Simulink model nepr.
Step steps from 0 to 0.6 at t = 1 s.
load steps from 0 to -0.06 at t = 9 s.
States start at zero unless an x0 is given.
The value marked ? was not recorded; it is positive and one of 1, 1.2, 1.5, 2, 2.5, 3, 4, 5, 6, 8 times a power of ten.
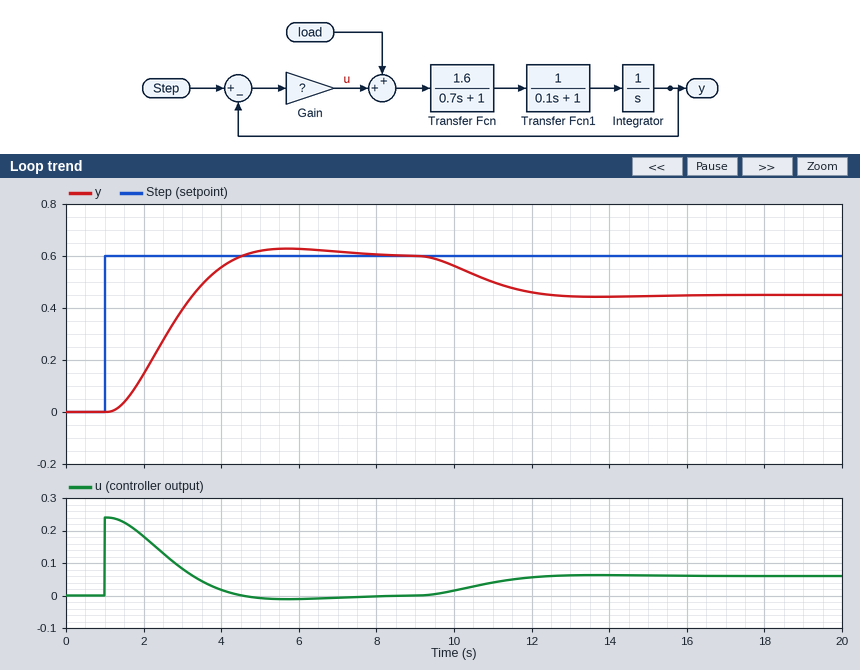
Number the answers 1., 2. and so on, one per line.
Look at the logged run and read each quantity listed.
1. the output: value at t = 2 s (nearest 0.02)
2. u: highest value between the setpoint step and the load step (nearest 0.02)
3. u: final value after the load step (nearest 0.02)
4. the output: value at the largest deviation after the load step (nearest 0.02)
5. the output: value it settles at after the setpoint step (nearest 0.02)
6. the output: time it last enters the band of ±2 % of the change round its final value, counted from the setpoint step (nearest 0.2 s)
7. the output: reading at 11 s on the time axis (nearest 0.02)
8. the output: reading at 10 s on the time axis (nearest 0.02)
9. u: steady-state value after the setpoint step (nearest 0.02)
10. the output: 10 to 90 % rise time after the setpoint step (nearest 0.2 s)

1. 0.14
2. 0.24
3. 0.06
4. 0.44
5. 0.60
6. 6.4 s
7. 0.50
8. 0.56
9. 0.00
10. 2.2 s
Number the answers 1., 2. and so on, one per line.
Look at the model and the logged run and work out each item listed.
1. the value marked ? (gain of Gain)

1. 0.4
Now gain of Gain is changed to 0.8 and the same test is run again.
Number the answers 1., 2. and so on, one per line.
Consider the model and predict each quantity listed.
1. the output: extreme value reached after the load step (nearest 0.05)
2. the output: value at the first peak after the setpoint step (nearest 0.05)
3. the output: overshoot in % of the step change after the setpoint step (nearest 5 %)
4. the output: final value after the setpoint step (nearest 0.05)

1. 0.50
2. 0.70
3. 20 %
4. 0.60
